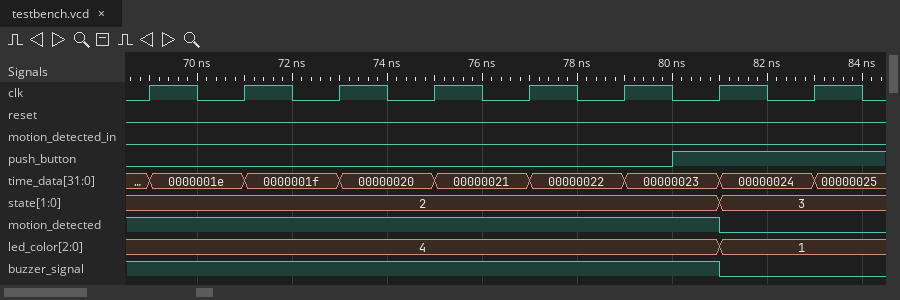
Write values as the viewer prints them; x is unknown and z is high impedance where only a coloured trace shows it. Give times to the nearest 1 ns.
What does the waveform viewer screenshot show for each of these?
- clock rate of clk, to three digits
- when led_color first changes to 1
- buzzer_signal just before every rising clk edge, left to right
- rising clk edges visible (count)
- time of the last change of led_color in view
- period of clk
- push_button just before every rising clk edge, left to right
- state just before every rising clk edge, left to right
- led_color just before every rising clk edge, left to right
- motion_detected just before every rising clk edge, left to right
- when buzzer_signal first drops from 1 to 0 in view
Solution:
500 MHz
81 ns
1 1 1 1 1 1 1 0
8
81 ns
2 ns
0 0 0 0 0 0 1 1
2, 2, 2, 2, 2, 2, 2, 3
4, 4, 4, 4, 4, 4, 4, 1
1 1 1 1 1 1 1 0
81 ns
